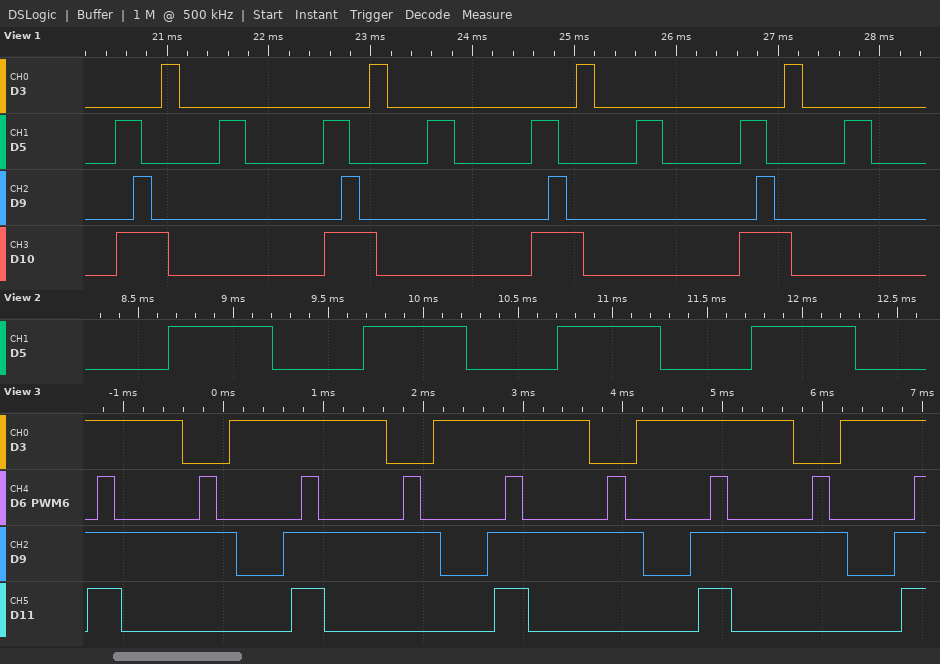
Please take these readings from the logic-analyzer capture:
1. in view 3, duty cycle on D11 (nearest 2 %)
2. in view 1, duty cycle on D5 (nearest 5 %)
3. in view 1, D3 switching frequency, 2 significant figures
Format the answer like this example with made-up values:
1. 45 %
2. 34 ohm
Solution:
1. 16 %
2. 25 %
3. 490 Hz
